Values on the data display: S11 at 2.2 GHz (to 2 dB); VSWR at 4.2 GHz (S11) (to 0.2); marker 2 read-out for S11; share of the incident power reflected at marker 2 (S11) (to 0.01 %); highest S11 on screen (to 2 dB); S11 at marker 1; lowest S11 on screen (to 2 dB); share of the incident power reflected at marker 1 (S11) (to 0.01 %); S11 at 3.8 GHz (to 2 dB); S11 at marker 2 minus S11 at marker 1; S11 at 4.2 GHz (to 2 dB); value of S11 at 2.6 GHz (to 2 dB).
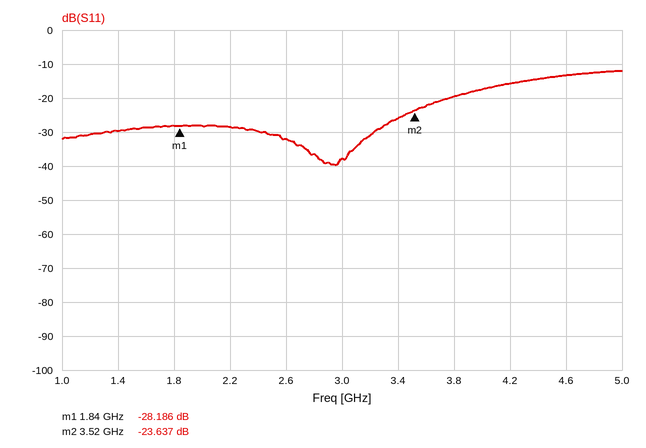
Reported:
-28 dB
1.4
-23.637 dB
0.43 %
-12 dB
-28.186 dB
-40 dB
0.15 %
-20 dB
4.549 dB
-16 dB
-32 dB
